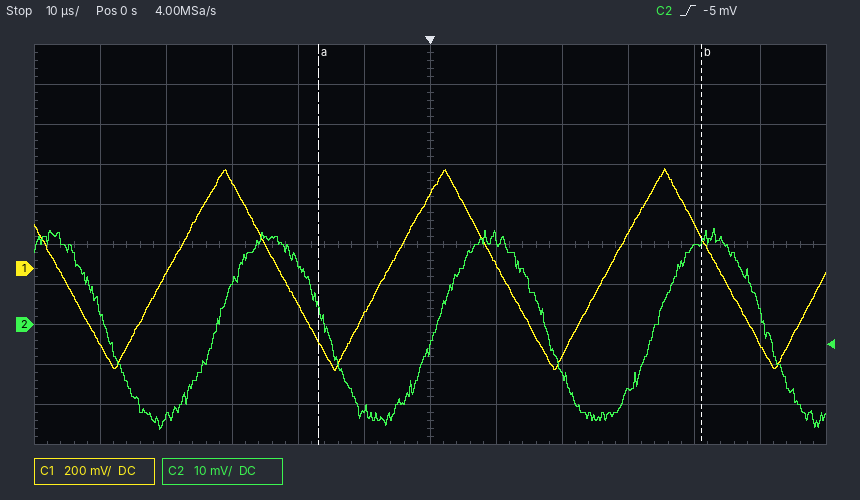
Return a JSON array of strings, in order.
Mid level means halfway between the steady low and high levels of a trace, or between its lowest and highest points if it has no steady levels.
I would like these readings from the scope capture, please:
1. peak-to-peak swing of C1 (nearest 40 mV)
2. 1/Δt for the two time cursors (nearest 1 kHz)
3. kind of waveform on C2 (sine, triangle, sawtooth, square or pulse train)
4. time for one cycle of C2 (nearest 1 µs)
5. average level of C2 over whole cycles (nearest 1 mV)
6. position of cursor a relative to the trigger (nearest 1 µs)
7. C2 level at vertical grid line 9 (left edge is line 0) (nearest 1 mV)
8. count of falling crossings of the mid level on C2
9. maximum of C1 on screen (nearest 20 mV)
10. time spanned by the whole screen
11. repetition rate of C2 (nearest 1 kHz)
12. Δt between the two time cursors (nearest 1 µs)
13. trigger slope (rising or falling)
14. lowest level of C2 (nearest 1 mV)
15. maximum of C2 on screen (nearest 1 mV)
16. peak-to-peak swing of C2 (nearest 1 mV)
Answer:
["1.00 V", "17 kHz", "sine", "33 µs", "-1 mV", "-17 µs", "-17 mV", "4", "500 mV", "120 µs", "30 kHz", "58 µs", "rising", "-26 mV", "24 mV", "50 mV"]
